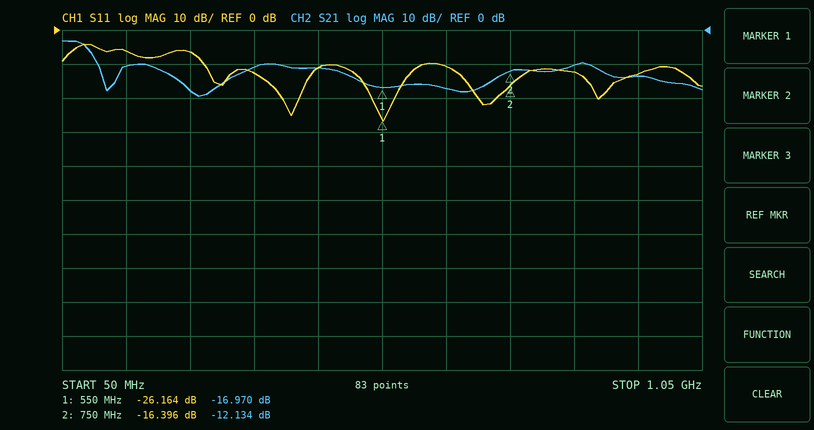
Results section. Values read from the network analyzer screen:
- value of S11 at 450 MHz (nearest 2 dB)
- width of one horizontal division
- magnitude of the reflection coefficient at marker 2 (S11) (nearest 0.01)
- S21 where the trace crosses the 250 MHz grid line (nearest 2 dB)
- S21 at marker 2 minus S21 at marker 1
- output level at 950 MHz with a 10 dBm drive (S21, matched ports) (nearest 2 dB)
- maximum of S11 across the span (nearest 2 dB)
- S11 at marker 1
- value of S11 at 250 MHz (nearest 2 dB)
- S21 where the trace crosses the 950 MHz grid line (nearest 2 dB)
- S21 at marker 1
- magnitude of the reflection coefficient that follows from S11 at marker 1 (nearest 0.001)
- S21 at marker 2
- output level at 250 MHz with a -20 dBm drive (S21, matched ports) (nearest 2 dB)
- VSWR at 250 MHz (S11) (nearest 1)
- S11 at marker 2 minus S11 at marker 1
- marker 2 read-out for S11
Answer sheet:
-12 dB
100 MHz
0.15
-18 dB
4.836 dB
-4 dBm
-4 dB
-26.164 dB
-6 dB
-14 dB
-16.970 dB
0.049
-12.134 dB
-38 dBm
3
9.768 dB
-16.396 dB
